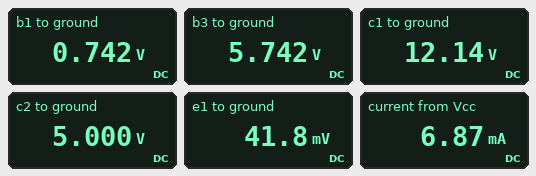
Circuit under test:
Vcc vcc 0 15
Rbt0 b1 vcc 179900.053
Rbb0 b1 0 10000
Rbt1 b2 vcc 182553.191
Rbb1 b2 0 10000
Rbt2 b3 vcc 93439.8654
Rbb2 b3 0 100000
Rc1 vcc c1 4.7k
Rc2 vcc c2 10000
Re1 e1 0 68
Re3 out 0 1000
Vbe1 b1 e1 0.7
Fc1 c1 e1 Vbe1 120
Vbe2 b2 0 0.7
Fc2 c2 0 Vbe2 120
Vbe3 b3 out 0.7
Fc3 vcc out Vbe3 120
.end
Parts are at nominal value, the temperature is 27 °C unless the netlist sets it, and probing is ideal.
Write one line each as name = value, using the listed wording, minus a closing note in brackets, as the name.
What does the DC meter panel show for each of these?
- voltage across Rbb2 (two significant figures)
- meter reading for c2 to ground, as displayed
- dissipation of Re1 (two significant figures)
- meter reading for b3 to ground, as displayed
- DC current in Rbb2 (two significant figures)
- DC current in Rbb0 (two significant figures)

voltage across Rbb2 = 5.7 V
meter reading for c2 to ground, as displayed = 5.000 V
dissipation of Re1 = 26 µW
meter reading for b3 to ground, as displayed = 5.742 V
DC current in Rbb2 = 57 µA
DC current in Rbb0 = 74 µA
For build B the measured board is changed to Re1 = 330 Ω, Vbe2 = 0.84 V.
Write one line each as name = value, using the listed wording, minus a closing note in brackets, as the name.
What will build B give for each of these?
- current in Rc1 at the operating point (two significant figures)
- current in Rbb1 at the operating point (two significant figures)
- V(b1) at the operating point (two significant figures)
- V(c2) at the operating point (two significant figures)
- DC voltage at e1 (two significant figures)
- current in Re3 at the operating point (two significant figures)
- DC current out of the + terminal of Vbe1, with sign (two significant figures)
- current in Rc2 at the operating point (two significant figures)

current in Rc1 at the operating point = 220 µA
current in Rbb1 at the operating point = 84 µA
V(b1) at the operating point = 770 mV
V(c2) at the operating point = 23 V
DC voltage at e1 = 73 mV
current in Re3 at the operating point = 5.0 mA
DC current out of the + terminal of Vbe1, with sign = -1.8 µA
current in Rc2 at the operating point = 770 µA
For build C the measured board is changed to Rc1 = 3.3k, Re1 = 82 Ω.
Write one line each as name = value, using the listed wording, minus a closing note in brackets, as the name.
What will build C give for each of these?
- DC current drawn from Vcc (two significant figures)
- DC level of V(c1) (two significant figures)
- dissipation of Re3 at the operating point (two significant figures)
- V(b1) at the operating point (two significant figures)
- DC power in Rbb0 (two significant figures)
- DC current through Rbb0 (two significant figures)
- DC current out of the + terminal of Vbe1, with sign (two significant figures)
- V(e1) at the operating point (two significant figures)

DC current drawn from Vcc = 6.8 mA
DC level of V(c1) = 13 V
dissipation of Re3 at the operating point = 25 mW
V(b1) at the operating point = 750 mV
DC power in Rbb0 = 56 µW
DC current through Rbb0 = 75 µA
DC current out of the + terminal of Vbe1, with sign = -4.6 µA
V(e1) at the operating point = 46 mV
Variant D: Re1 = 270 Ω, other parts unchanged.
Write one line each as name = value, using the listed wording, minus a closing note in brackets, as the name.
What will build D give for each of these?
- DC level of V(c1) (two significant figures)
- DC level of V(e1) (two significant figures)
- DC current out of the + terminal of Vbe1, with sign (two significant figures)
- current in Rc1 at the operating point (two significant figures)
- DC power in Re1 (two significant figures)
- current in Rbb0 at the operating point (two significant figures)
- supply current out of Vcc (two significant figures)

DC level of V(c1) = 14 V
DC level of V(e1) = 70 mV
DC current out of the + terminal of Vbe1, with sign = -2.1 µA
current in Rc1 at the operating point = 260 µA
DC power in Re1 = 18 µW
current in Rbb0 at the operating point = 77 µA
supply current out of Vcc = 6.5 mA
